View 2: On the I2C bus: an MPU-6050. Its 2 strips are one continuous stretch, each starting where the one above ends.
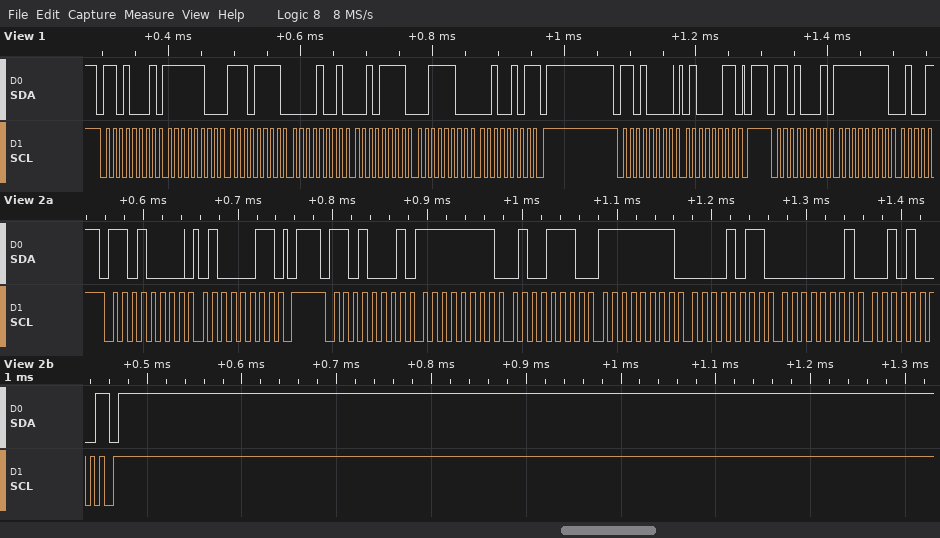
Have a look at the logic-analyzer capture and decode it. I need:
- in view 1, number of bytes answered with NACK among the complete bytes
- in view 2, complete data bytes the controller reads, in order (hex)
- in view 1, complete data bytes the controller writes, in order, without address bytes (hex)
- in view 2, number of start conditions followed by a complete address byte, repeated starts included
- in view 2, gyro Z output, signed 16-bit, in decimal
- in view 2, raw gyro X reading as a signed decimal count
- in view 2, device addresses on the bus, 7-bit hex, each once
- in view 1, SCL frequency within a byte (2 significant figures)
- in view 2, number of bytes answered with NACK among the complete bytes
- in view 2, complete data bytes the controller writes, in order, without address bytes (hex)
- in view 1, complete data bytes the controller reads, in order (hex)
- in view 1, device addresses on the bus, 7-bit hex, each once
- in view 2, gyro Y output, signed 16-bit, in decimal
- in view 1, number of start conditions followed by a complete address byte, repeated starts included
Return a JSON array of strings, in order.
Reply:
["1", "FF 4E FF 0B 01 28", "43", "2", "296", "-178", "0x68", "100 kHz", "1", "43", "FC EF 09 2F 3C 25 FF", "0x68", "-245", "3"]
